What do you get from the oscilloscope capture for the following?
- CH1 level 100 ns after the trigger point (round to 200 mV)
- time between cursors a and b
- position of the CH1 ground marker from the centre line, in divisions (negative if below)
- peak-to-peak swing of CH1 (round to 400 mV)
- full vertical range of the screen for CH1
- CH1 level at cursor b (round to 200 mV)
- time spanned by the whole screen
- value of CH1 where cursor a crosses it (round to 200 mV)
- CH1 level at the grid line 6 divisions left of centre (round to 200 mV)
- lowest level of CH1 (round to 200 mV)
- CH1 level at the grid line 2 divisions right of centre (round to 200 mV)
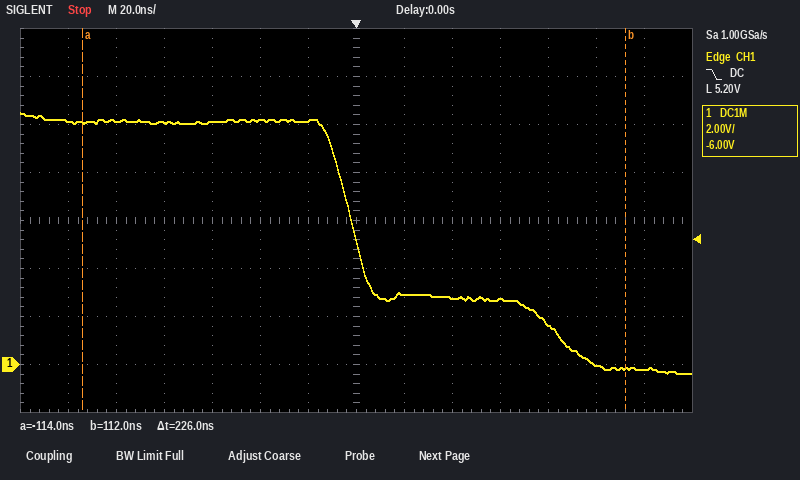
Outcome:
0.0 V
226 ns
-3.0 div
10.8 V
16 V
-200 mV
280 ns
10.0 V
10.2 V
-400 mV
2.8 V
